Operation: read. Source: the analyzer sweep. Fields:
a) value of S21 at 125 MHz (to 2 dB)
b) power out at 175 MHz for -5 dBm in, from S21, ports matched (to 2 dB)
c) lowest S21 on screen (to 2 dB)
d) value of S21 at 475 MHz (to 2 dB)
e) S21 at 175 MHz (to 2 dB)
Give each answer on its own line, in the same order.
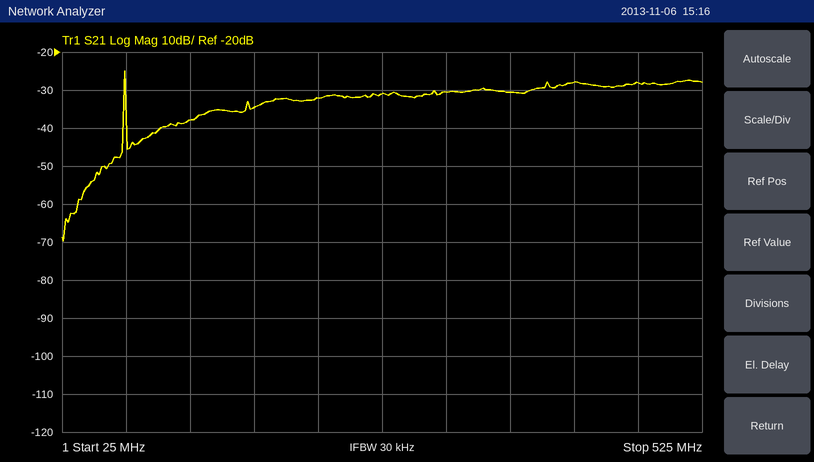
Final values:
-38 dB
-40 dBm
-70 dB
-28 dB
-34 dB
